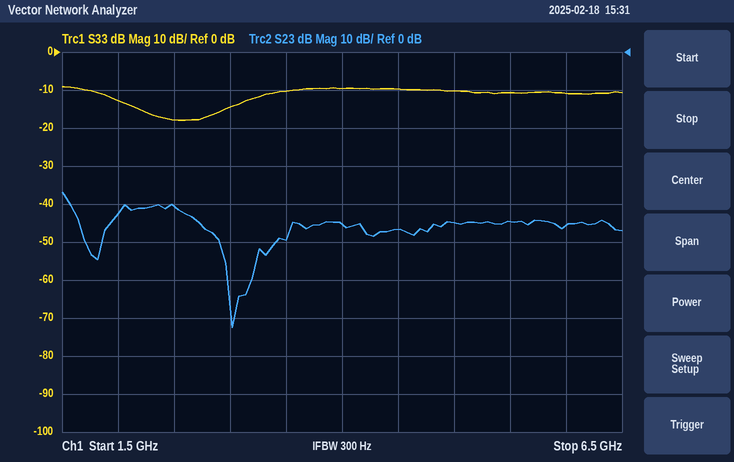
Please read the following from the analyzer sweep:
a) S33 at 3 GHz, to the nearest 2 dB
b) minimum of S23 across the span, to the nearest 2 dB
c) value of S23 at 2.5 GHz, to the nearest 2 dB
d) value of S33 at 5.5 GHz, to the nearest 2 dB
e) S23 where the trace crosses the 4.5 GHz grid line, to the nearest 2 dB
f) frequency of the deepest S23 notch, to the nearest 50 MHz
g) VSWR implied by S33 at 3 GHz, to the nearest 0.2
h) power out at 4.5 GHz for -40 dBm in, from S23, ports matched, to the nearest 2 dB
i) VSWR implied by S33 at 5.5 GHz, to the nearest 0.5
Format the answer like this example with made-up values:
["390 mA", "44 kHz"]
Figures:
["-14 dB", "-72 dB", "-40 dB", "-10 dB", "-46 dB", "3.00 GHz", "1.4", "-86 dBm", "2.0"]
